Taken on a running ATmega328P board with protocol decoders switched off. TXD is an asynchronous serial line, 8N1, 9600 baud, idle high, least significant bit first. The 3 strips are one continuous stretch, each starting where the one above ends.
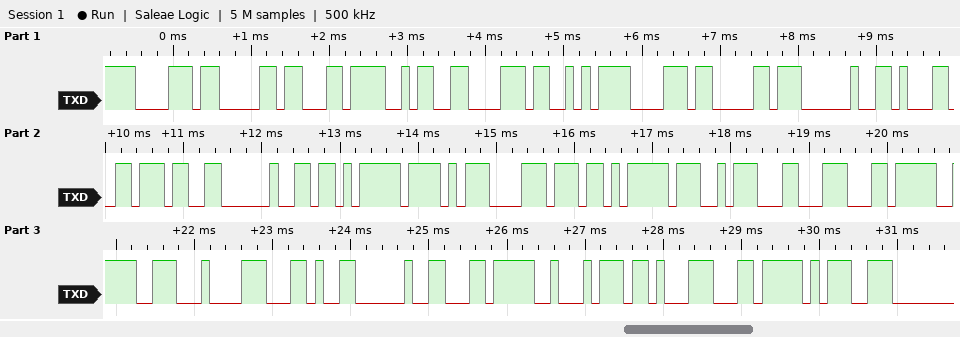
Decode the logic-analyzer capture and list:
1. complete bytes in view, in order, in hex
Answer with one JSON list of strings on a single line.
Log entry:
["0xB8 0xB0 0xEC 0x9A 0xB8 0xEA 0xB8 0xB0 0x20 0x31 0x37 0x20 0xEB 0xAF 0xB8 0xEB 0xA7 0x8C 0xEC 0x9E 0x84 0x2C 0x20 0xEC 0xA2 0x8B 0xEC 0x9D"]
